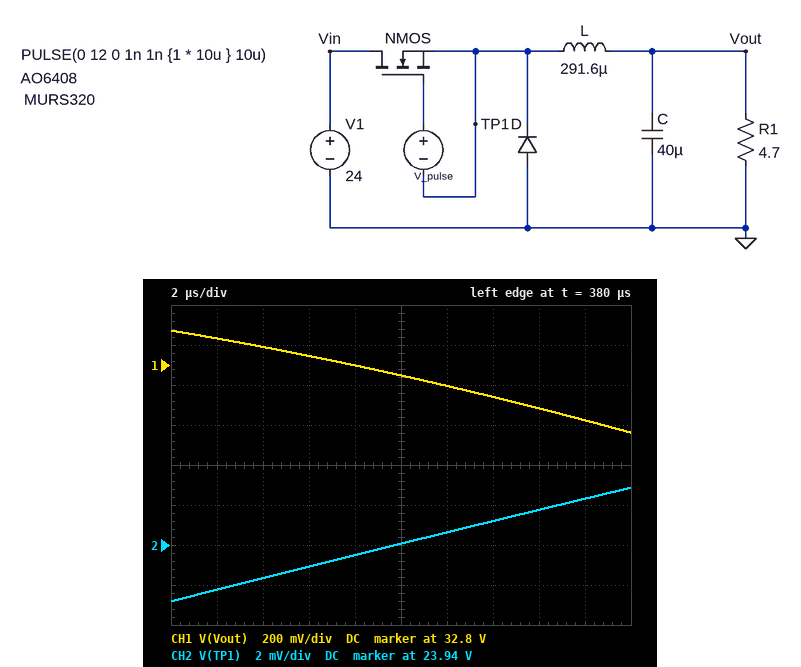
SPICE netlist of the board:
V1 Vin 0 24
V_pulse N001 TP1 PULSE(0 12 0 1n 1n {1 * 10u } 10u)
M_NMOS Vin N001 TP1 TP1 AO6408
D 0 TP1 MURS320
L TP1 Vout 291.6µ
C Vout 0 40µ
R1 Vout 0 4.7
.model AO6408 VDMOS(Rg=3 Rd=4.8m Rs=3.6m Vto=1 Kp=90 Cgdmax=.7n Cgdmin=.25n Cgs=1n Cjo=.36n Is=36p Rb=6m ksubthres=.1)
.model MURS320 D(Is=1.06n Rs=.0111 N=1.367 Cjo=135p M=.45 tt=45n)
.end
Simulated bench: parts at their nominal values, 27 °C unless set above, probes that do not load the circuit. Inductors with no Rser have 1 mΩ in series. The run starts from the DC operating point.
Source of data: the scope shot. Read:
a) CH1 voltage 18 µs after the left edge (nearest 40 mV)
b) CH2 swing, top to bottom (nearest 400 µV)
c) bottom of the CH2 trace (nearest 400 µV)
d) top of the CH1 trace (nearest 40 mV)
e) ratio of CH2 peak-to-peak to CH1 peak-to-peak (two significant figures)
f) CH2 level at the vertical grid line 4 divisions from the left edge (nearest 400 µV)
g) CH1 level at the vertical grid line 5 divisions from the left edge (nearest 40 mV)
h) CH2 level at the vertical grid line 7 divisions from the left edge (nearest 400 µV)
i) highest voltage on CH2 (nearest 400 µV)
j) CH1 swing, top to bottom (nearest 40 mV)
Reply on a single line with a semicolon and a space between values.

32.52 V; 5.6 mV; 23.9412 V; 32.96 V; 0.011; 23.9436 V; 32.76 V; 23.9452 V; 23.9468 V; 520 mV
